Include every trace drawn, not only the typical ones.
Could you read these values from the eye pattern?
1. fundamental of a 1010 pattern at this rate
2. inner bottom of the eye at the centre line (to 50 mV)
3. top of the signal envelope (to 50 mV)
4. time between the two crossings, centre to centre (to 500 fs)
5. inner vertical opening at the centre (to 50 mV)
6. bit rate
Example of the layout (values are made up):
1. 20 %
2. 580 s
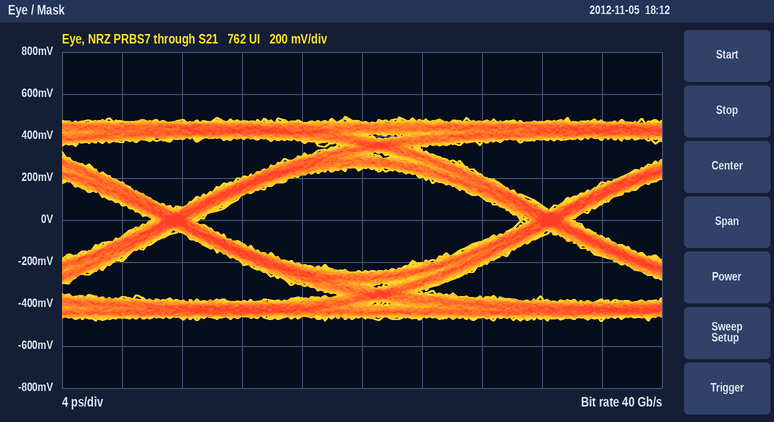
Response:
1. 20 GHz
2. -250 mV
3. 500 mV
4. 25.0 ps
5. 500 mV
6. 40 Gb/s
